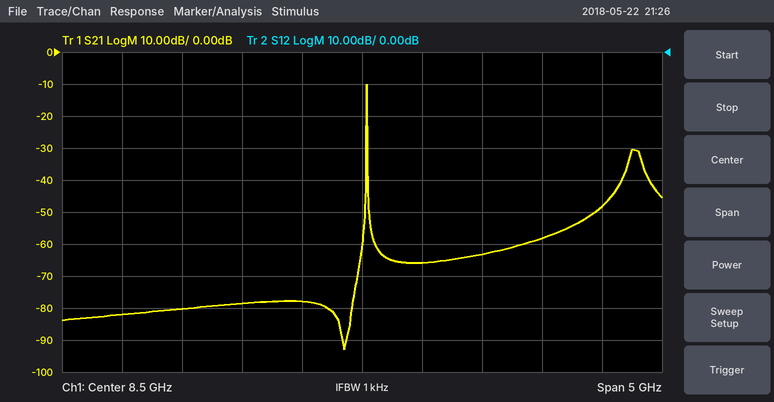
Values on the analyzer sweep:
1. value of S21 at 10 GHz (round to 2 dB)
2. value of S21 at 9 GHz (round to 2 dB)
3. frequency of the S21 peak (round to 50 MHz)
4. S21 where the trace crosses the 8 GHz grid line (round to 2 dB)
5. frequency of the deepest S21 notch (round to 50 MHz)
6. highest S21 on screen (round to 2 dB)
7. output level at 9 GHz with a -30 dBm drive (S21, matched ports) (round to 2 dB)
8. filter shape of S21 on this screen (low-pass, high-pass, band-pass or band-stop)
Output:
-58 dB
-66 dB
8.55 GHz
-78 dB
8.35 GHz
-10 dB
-96 dBm
band-pass
